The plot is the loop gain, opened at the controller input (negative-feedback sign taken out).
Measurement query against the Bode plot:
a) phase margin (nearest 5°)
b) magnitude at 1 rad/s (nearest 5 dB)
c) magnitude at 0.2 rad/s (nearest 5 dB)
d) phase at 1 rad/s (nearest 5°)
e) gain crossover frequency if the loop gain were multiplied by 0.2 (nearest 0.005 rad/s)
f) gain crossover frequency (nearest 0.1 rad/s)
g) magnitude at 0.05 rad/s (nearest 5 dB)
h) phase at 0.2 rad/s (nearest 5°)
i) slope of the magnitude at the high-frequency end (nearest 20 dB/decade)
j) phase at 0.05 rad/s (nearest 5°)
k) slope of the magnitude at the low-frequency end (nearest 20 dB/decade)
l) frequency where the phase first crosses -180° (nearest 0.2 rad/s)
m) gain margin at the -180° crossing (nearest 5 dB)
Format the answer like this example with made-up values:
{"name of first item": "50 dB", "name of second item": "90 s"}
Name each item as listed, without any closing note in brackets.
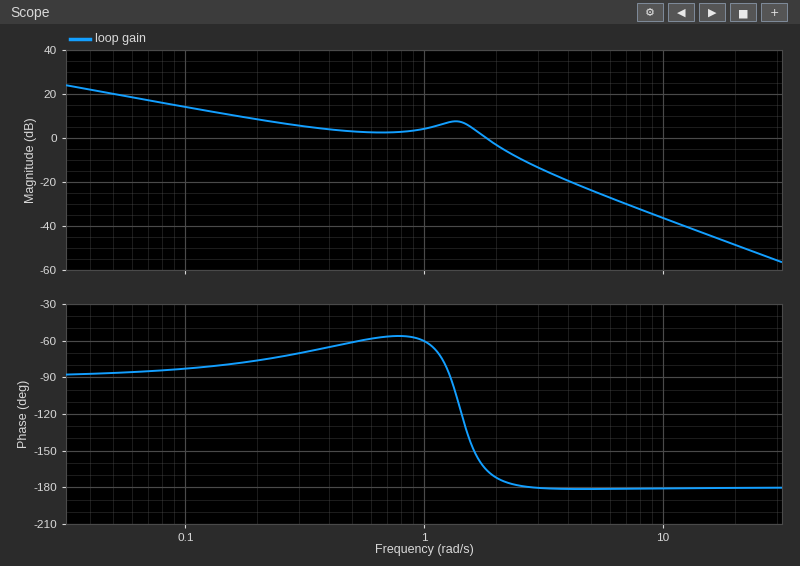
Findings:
{"phase margin": "15°", "magnitude at 1 rad/s": "5 dB", "magnitude at 0.2 rad/s": "10 dB", "phase at 1 rad/s": "-60°", "gain crossover frequency if the loop gain were multiplied by 0.2": "0.100 rad/s", "gain crossover frequency": "1.8 rad/s", "magnitude at 0.05 rad/s": "20 dB", "phase at 0.2 rad/s": "-75°", "slope of the magnitude at the high-frequency end": "-40 dB/decade", "phase at 0.05 rad/s": "-85°", "slope of the magnitude at the low-frequency end": "-20 dB/decade", "frequency where the phase first crosses -180°": "2.8 rad/s", "gain margin at the -180° crossing": "10 dB"}
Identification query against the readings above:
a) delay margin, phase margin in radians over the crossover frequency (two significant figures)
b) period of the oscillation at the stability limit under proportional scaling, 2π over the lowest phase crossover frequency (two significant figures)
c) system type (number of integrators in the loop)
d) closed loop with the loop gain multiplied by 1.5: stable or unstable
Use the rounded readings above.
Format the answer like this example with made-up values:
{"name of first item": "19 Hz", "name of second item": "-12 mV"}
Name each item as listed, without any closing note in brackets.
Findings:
{"delay margin, phase margin in radians over the crossover frequency": "0.15 s", "period of the oscillation at the stability limit under proportional scaling, 2π over the lowest phase crossover frequency": "2.2 s", "system type": "1", "closed loop with the loop gain multiplied by 1.5: stable or unstable": "stable"}
